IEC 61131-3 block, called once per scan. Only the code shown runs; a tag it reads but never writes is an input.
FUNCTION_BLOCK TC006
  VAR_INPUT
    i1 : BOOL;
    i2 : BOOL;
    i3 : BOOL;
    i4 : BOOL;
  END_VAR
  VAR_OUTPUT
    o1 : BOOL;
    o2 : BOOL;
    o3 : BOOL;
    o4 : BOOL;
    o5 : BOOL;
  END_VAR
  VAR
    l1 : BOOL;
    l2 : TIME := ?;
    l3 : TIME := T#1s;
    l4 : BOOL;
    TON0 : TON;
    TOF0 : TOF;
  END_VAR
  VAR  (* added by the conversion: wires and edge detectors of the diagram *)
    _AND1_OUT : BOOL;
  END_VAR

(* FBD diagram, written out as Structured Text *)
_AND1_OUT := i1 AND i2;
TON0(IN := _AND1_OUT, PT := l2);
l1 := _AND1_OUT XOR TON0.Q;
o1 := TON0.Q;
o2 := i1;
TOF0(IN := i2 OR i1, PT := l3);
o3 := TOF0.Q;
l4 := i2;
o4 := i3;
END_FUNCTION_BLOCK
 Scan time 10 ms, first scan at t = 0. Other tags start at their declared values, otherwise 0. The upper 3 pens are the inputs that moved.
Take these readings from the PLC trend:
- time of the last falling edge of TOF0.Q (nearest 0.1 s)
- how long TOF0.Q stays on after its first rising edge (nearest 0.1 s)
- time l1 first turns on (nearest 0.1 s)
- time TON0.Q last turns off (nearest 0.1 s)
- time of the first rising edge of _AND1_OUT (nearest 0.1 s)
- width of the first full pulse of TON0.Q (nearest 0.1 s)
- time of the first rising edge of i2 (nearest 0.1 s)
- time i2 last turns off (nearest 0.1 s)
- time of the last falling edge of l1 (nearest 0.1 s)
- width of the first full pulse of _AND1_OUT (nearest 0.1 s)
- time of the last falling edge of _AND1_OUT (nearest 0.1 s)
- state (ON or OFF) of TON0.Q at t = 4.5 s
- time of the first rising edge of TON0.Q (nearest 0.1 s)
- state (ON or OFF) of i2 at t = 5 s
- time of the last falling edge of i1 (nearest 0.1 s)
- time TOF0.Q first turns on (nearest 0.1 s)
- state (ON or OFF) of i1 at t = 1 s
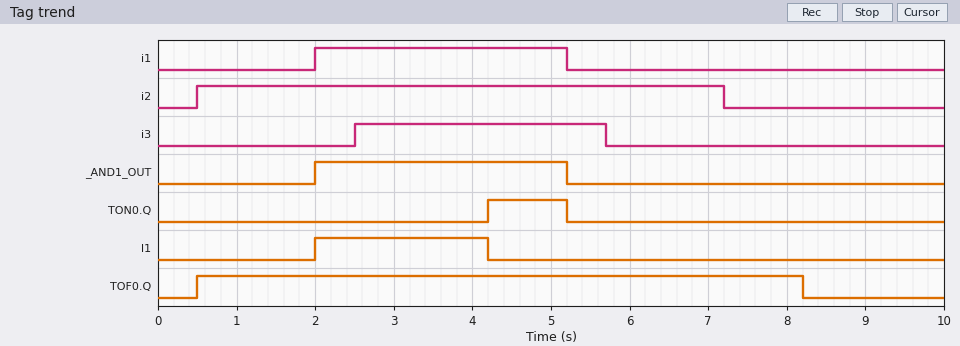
8.2 s
7.7 s
2.0 s
5.2 s
2.0 s
1.0 s
0.5 s
7.2 s
4.2 s
3.2 s
5.2 s
ON
4.2 s
ON
5.2 s
0.5 s
OFF
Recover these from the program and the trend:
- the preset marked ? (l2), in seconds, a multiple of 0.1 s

2.2 s
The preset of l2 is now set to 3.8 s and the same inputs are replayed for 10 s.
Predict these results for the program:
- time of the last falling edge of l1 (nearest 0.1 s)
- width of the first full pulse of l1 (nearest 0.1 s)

5.2 s
3.2 s
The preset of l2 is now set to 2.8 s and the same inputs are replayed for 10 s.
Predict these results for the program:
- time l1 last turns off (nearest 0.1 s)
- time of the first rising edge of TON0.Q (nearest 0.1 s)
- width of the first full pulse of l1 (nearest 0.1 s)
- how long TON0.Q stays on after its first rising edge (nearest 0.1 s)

4.8 s
4.8 s
2.8 s
0.4 s
